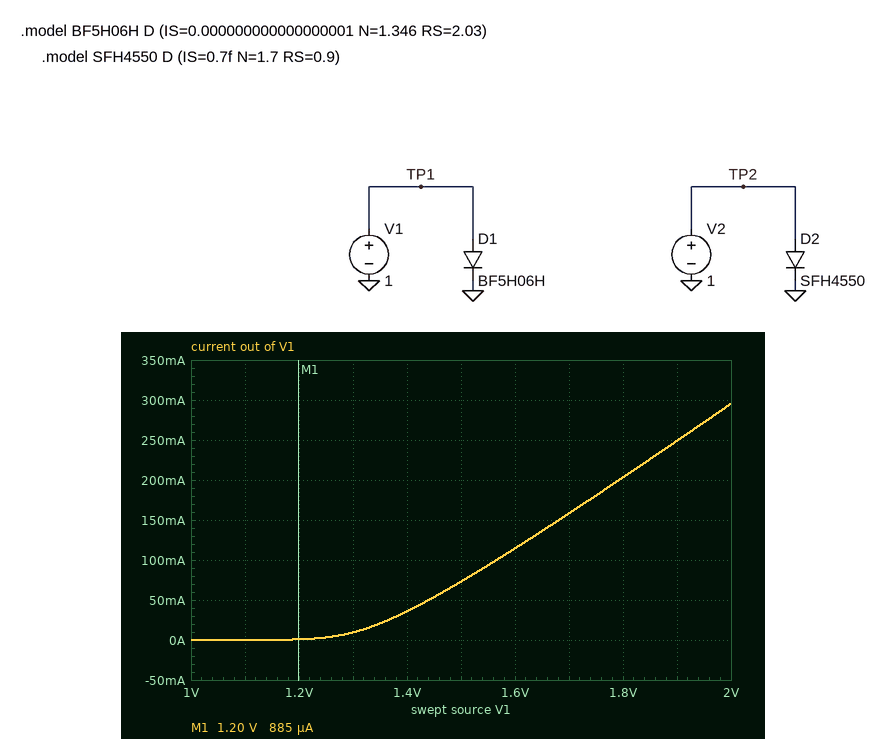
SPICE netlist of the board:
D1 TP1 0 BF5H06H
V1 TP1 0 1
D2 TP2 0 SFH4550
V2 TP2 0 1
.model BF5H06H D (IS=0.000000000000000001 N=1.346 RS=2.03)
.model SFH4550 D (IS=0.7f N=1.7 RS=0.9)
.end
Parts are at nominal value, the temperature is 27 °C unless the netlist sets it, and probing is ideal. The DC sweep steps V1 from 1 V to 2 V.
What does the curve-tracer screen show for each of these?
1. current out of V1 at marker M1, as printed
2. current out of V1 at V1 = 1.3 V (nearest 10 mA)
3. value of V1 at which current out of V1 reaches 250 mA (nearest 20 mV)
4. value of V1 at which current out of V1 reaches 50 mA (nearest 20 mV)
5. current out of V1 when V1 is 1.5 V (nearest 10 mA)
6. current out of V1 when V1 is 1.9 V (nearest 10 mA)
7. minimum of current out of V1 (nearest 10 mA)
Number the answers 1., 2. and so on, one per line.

1. 885 µA
2. 10 mA
3. 1.90 V
4. 1.44 V
5. 70 mA
6. 250 mA
7. 0 A
